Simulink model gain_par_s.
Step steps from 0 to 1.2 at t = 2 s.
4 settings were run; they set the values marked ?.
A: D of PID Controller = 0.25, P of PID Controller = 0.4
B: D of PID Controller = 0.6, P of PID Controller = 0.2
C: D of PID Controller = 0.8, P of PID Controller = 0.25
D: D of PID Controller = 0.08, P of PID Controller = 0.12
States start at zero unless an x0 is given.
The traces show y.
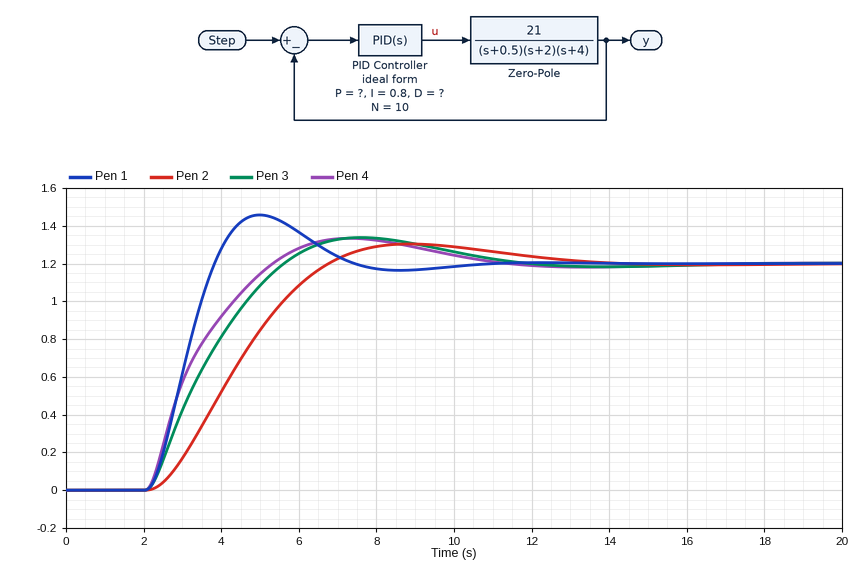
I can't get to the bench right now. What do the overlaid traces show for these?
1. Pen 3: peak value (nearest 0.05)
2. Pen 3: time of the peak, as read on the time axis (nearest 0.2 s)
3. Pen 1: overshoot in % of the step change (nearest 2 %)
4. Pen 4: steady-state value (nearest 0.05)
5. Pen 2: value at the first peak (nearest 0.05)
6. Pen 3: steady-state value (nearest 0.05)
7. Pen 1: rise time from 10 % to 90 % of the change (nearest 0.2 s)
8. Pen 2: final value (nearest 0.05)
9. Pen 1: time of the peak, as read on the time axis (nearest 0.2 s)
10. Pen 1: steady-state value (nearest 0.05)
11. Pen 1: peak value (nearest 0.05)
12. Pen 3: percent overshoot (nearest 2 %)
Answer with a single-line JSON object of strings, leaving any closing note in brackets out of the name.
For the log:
{"Pen 3: peak value": "1.35", "Pen 3: time of the peak, as read on the time axis": "7.6 s", "Pen 1: overshoot in % of the step change": "22 %", "Pen 4: steady-state value": "1.20", "Pen 2: value at the first peak": "1.30", "Pen 3: steady-state value": "1.20", "Pen 1: rise time from 10 % to 90 % of the change": "1.2 s", "Pen 2: final value": "1.20", "Pen 1: time of the peak, as read on the time axis": "5.0 s", "Pen 1: steady-state value": "1.20", "Pen 1: peak value": "1.45", "Pen 3: percent overshoot": "12 %"}
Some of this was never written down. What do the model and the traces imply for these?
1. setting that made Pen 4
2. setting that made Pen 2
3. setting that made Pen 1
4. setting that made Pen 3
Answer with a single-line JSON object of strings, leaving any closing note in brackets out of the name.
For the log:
{"setting that made Pen 4": "C", "setting that made Pen 2": "D", "setting that made Pen 1": "A", "setting that made Pen 3": "B"}
